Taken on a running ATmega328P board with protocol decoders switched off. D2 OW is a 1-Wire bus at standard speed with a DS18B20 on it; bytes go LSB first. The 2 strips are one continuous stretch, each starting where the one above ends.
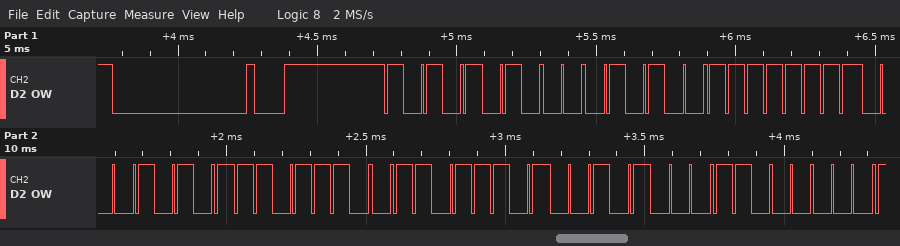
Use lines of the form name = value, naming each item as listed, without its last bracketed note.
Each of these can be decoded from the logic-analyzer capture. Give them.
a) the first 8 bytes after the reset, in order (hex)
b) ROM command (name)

the first 8 bytes after the reset, in order = 55 28 FF A8 3B BB 14 03
ROM command = Match ROM
